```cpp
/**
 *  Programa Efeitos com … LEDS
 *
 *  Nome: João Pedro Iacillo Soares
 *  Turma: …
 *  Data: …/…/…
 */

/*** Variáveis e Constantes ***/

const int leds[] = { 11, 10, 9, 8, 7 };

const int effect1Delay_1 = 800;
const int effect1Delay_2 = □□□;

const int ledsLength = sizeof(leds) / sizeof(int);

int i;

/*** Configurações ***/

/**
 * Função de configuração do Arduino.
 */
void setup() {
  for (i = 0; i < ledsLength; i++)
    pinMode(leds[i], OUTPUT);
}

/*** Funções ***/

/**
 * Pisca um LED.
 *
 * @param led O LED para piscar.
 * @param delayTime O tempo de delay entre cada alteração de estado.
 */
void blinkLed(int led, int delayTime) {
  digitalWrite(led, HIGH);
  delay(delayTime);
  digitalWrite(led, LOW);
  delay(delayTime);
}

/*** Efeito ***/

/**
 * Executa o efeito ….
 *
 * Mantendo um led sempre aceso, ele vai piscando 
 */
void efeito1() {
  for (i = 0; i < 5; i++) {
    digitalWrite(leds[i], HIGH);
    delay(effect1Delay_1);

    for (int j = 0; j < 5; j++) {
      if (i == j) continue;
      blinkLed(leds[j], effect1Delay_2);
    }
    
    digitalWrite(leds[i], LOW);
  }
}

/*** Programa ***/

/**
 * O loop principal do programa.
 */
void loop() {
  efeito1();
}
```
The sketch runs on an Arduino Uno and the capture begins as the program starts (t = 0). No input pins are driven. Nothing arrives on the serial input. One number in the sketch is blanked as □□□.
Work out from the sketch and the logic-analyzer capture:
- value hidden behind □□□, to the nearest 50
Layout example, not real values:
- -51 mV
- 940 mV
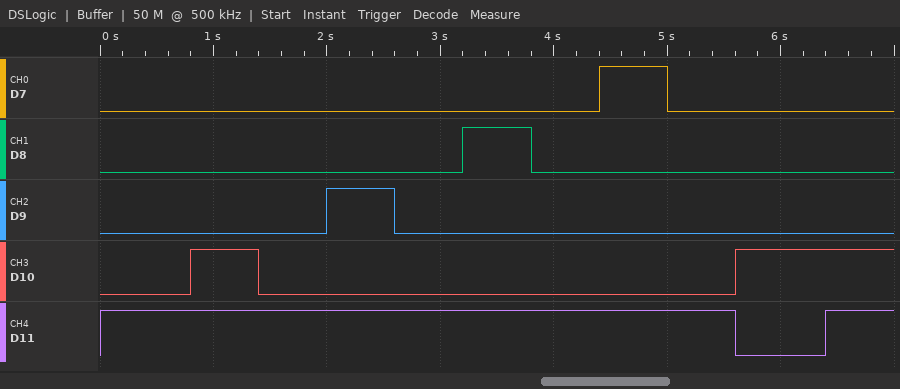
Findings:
- 600
